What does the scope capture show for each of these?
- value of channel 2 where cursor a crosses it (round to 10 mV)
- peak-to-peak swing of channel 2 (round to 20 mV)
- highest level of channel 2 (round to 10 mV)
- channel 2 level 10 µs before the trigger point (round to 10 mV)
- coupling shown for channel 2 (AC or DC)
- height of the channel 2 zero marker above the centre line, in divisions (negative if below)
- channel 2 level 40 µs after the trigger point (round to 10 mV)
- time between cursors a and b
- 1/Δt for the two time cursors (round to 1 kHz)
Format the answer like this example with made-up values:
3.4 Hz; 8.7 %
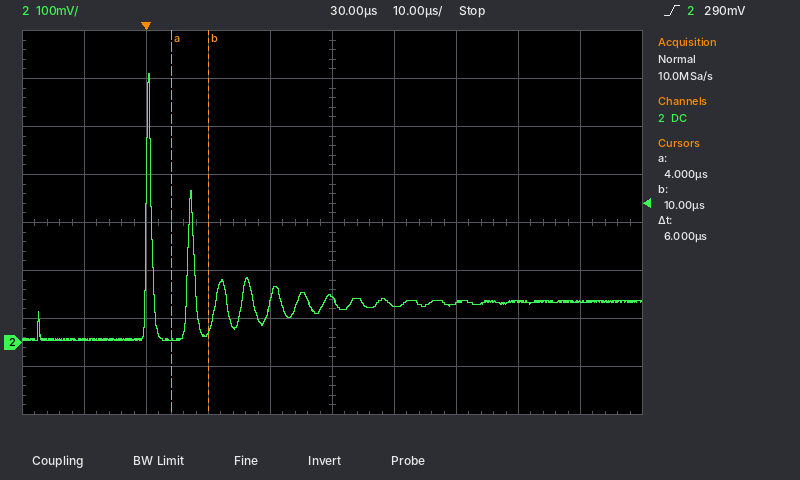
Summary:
10 mV; 560 mV; 560 mV; 10 mV; DC; -2.5 div; 80 mV; 6 µs; 167 kHz
